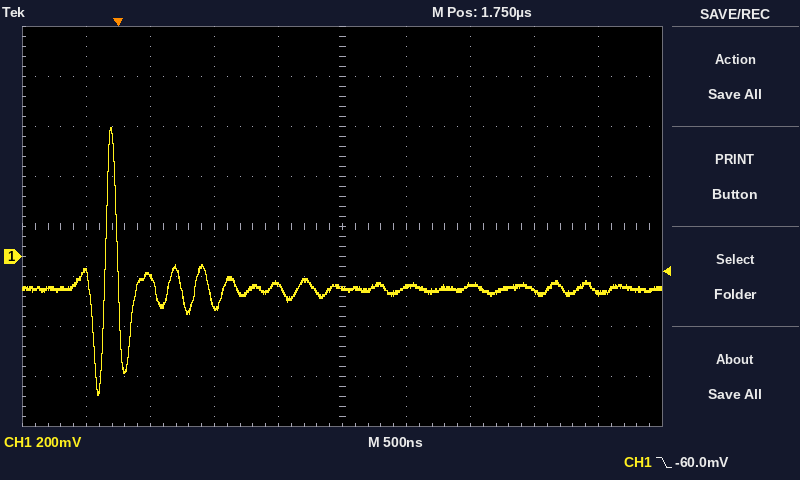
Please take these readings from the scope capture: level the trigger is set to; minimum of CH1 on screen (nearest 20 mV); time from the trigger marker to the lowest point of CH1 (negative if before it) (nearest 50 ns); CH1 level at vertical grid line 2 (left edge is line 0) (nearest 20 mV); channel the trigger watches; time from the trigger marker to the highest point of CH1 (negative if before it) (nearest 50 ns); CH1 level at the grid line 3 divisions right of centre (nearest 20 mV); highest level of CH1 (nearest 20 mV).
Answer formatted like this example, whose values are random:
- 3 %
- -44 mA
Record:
- -60.0 mV
- -560 mV
- -150 ns
- -80 mV
- CH1
- -50 ns
- -140 mV
- 520 mV
